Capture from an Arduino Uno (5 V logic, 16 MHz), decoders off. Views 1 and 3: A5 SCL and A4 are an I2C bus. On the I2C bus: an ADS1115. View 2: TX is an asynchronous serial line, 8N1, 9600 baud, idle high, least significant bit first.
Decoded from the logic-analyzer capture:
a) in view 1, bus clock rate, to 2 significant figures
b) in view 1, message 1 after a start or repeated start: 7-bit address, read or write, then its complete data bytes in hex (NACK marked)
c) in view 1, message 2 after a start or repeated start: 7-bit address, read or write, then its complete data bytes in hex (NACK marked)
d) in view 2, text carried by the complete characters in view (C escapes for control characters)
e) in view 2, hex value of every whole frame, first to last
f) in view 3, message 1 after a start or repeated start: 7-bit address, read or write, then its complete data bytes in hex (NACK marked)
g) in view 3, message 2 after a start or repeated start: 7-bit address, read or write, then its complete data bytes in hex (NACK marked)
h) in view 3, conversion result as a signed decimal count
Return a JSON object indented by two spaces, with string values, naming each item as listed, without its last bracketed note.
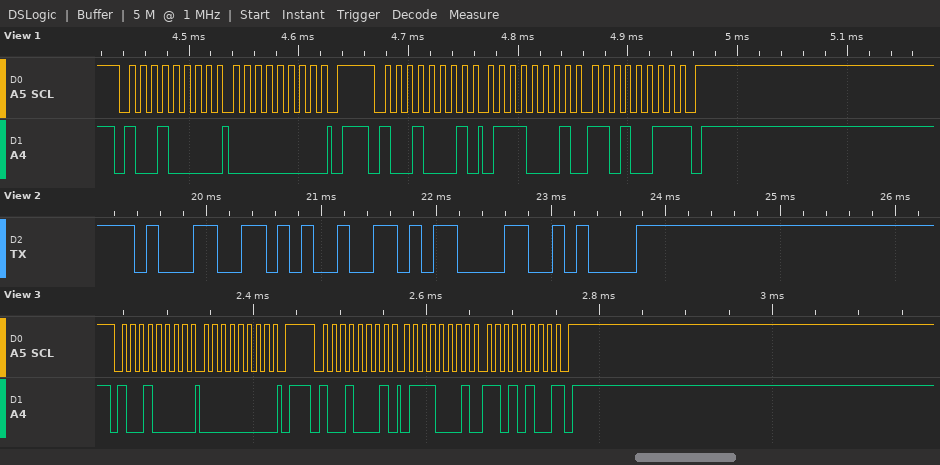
{
  "in view 1, bus clock rate, to 2 significant figures": "100 kHz",
  "in view 1, message 1 after a start or repeated start: 7-bit address, read or write, then its complete data bytes in hex": "0x48 write: 00",
  "in view 1, message 2 after a start or repeated start: 7-bit address, read or write, then its complete data bytes in hex": "0x48 read: 71 D3 NACK",
  "in view 2, text carried by the complete characters in view": "\"1%\\r\\n\"",
  "in view 2, hex value of every whole frame, first to last": "31 25 0D 0A",
  "in view 3, message 1 after a start or repeated start: 7-bit address, read or write, then its complete data bytes in hex": "0x48 write: 00",
  "in view 3, message 2 after a start or repeated start: 7-bit address, read or write, then its complete data bytes in hex": "0x48 read: 71 D4 NACK",
  "in view 3, conversion result as a signed decimal count": "29140"
}
